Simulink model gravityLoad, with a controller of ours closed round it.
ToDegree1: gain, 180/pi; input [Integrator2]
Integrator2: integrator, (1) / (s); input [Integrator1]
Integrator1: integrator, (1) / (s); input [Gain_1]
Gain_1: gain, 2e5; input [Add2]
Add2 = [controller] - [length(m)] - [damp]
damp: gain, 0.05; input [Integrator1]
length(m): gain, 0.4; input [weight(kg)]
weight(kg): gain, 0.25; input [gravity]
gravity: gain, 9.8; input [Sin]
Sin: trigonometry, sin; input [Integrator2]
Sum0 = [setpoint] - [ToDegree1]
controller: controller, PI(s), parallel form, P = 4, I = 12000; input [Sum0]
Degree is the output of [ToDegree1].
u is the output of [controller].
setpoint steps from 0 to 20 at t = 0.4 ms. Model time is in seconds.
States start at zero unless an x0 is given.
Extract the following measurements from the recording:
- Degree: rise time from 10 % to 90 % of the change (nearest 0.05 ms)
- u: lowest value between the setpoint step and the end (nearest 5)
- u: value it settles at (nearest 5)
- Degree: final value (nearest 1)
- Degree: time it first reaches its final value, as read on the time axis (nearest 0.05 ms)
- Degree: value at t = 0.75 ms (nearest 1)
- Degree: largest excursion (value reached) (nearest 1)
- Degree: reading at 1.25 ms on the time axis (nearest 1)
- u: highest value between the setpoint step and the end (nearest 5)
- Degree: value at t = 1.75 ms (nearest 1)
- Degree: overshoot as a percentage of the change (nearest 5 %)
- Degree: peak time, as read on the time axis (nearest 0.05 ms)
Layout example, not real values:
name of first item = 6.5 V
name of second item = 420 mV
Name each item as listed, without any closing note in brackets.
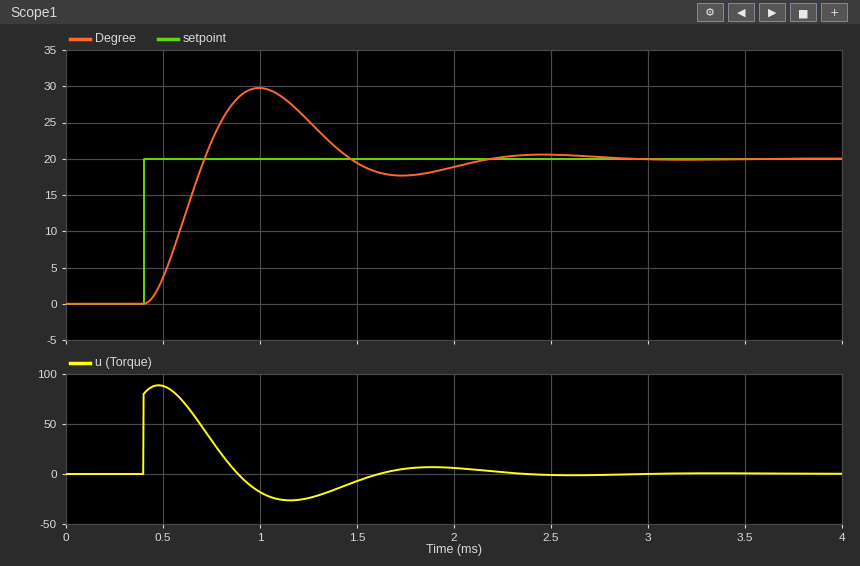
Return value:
Degree: rise time from 10 % to 90 % of the change = 0.20 ms
u: lowest value between the setpoint step and the end = -25
u: value it settles at = 0
Degree: final value = 20
Degree: time it first reaches its final value, as read on the time axis = 0.70 ms
Degree: value at t = 0.75 ms = 22
Degree: largest excursion (value reached) = 30
Degree: reading at 1.25 ms on the time axis = 25
u: highest value between the setpoint step and the end = 90
Degree: value at t = 1.75 ms = 18
Degree: overshoot as a percentage of the change = 50 %
Degree: peak time, as read on the time axis = 1.00 ms
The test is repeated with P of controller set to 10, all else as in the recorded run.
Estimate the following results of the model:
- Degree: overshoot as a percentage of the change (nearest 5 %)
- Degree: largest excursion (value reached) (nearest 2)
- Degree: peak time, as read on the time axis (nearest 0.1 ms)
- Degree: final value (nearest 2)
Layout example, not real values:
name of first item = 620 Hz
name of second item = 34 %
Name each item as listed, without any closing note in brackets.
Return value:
Degree: overshoot as a percentage of the change = 35 %
Degree: largest excursion (value reached) = 26
Degree: peak time, as read on the time axis = 0.7 ms
Degree: final value = 20
